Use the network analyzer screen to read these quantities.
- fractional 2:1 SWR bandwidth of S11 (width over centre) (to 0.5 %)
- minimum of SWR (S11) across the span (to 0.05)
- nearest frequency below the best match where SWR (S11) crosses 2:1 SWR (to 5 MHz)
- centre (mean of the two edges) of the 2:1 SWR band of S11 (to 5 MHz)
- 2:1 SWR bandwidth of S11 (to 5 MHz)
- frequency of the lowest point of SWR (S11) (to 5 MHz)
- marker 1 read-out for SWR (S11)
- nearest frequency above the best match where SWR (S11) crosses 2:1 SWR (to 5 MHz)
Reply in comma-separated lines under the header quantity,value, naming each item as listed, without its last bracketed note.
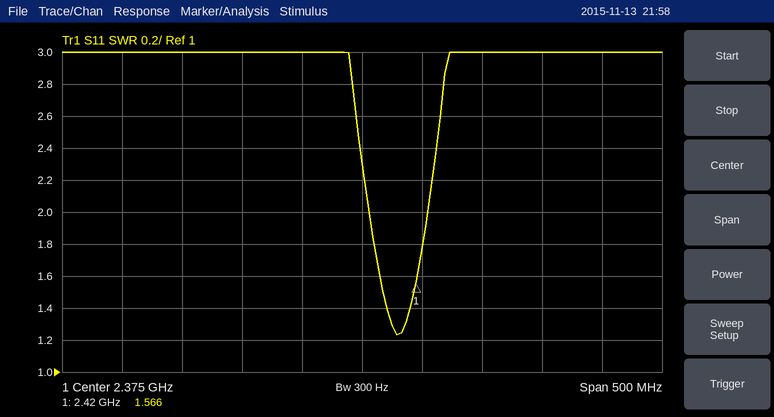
quantity,value
fractional 2:1 SWR bandwidth of S11 (width over centre),2.0 %
minimum of SWR (S11) across the span,1.25
nearest frequency below the best match where SWR (S11) crosses 2:1 SWR,2.380 GHz
centre (mean of the two edges) of the 2:1 SWR band of S11,2.405 GHz
2:1 SWR bandwidth of S11,50 MHz
frequency of the lowest point of SWR (S11),2.405 GHz
marker 1 read-out for SWR,1.566
nearest frequency above the best match where SWR (S11) crosses 2:1 SWR,2.430 GHz
